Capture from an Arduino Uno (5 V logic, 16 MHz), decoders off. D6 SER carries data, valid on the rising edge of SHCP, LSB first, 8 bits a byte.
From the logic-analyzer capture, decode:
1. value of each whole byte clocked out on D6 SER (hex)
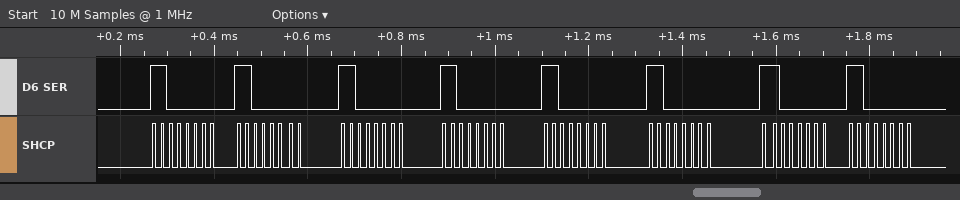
0x03 0x03 0x03 0x03 0x03 0x03 0x03 0x03
